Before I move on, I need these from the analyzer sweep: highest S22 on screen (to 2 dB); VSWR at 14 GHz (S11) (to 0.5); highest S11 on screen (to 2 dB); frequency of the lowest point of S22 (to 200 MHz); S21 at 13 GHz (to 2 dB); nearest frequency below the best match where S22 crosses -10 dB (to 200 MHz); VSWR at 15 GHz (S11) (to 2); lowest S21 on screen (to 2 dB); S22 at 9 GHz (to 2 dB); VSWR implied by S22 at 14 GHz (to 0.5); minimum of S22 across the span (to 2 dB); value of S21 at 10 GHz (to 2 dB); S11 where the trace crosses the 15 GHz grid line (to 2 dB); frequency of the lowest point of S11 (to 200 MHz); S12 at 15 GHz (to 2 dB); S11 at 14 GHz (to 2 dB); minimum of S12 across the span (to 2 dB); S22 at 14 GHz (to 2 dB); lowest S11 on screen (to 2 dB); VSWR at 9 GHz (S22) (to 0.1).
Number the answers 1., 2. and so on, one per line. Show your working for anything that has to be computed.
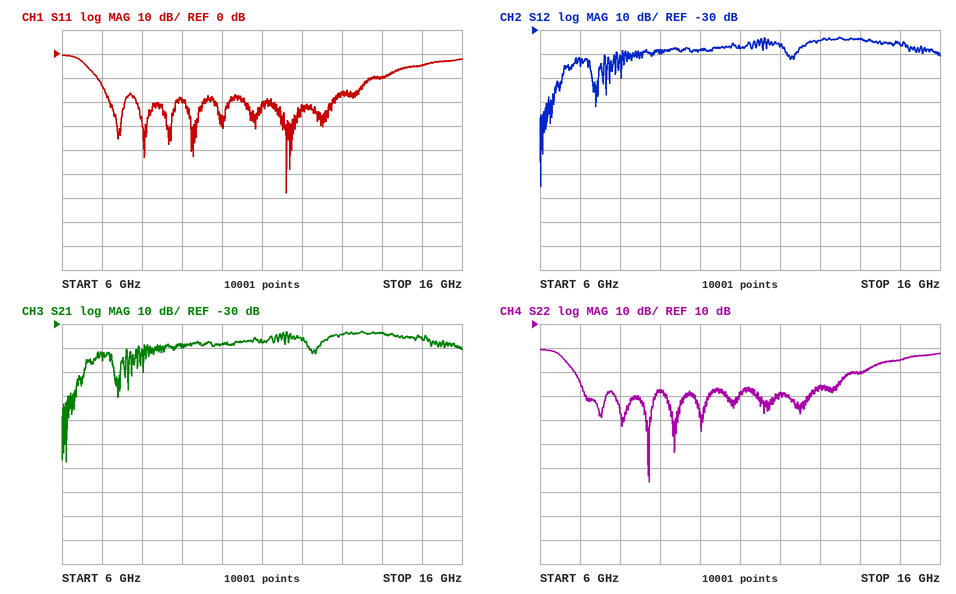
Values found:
1. 0 dB
2. |Γ| = 10^(-10/20) = 0.3162; VSWR = (1 + 0.3162)/(1 − 0.3162) ≈ 1.92, so 2.0 to the nearest 0.5
3. 0 dB
4. 8.8 GHz
5. -34 dB
6. 6.8 GHz
7. |Γ| = 10^(-4/20) = 0.6310; VSWR = (1 + 0.6310)/(1 − 0.6310) ≈ 4
8. -88 dB
9. -18 dB
10. |Γ| = 10^(-10/20) = 0.3162; VSWR = (1 + 0.3162)/(1 − 0.3162) ≈ 1.92, so 2.0 to the nearest 0.5
11. -56 dB
12. -38 dB
13. -4 dB
14. 11.6 GHz
15. -36 dB
16. -10 dB
17. -96 dB
18. -10 dB
19. -58 dB
20. |Γ| = 10^(-18/20) = 0.1259; VSWR = (1 + 0.1259)/(1 − 0.1259) ≈ 1.3
